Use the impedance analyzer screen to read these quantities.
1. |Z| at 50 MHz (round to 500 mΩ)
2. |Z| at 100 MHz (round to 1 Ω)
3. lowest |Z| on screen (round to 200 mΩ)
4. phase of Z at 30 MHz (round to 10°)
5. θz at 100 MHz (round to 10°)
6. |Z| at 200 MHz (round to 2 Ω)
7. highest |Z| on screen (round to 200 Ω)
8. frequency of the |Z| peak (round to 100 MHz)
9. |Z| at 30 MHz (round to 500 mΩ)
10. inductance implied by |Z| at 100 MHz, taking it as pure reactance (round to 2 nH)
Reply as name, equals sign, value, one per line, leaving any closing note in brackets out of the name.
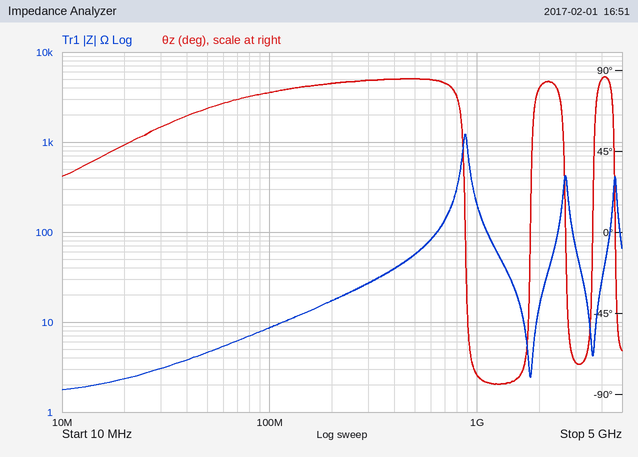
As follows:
|Z| at 50 MHz = 4.5 Ω
|Z| at 100 MHz = 9 Ω
lowest |Z| on screen = 1.8 Ω
phase of Z at 30 MHz = 60°
θz at 100 MHz = 80°
|Z| at 200 MHz = 18 Ω
highest |Z| on screen = 1.2 kΩ
frequency of the |Z| peak = 900 MHz
|Z| at 30 MHz = 3.0 Ω
inductance implied by |Z| at 100 MHz, taking it as pure reactance = 14 nH
